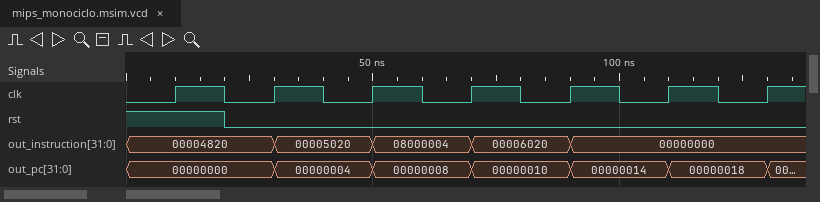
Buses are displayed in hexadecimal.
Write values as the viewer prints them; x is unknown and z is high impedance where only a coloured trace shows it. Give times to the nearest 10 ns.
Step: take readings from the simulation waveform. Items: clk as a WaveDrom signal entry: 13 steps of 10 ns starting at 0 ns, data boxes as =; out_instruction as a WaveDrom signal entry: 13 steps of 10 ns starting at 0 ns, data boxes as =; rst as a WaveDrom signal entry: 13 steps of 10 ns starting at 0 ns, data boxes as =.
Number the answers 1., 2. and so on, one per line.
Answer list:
1. {name: 'clk', wave: '0101010101010'}
2. {name: 'out_instruction', wave: '=..=.=.=.=...', data: '00004820 00005020 08000004 00006020 00000000'}
3. {name: 'rst', wave: '1.0..........'}
